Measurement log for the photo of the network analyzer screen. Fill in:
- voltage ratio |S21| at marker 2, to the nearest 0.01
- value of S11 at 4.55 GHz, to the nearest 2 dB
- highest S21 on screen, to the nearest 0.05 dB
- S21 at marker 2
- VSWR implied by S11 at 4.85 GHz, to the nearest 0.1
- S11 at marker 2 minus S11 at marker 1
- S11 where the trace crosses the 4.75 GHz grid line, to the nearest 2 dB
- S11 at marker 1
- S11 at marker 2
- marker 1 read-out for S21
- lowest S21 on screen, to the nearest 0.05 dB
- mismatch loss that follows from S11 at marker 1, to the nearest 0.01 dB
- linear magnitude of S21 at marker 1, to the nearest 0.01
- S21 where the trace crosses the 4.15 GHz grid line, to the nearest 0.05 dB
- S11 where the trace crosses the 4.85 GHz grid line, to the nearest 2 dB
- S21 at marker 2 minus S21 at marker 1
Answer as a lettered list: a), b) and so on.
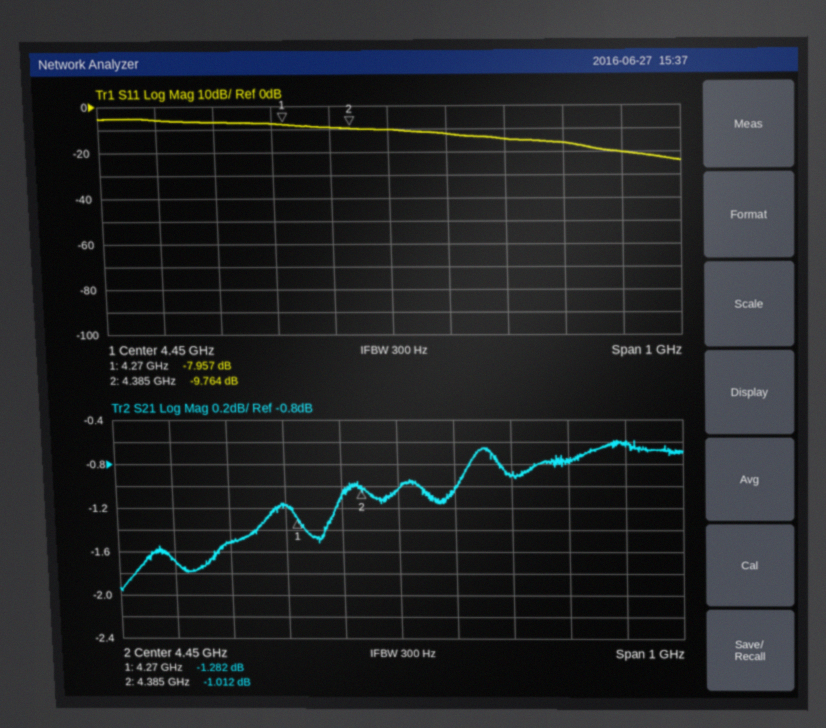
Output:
a) 0.89
b) -12 dB
c) -0.60 dB
d) -1.012 dB
e) 1.2
f) -1.807 dB
g) -16 dB
h) -7.957 dB
i) -9.764 dB
j) -1.282 dB
k) -1.95 dB
l) 0.76 dB
m) 0.86
n) -1.50 dB
o) -20 dB
p) 0.270 dB
